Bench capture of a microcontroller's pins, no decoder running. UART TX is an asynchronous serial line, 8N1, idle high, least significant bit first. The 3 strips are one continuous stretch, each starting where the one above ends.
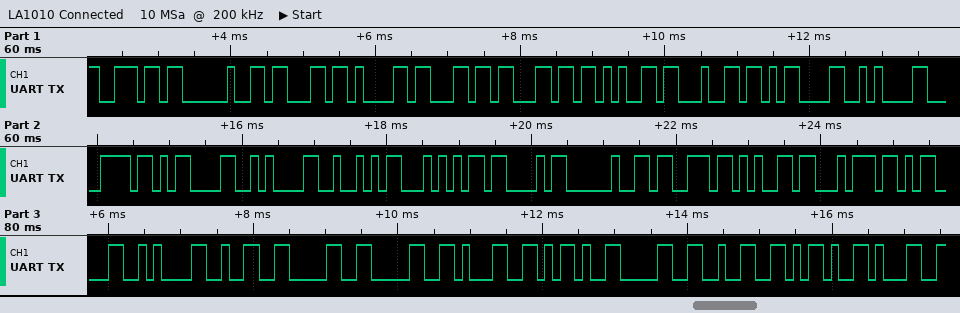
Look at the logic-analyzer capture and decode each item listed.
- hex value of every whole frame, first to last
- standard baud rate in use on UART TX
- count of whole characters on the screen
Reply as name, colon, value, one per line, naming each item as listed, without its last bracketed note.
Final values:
hex value of every whole frame, first to last: 6E 20 63 61 6C 6C 65 64 0D 0A 78 0D 0A 52 54 43 20 73 65 74 0D 0A 32 30 30 31 2D 30 32 2D 31
standard baud rate in use on UART TX: 9600 baud
count of whole characters on the screen: 31
